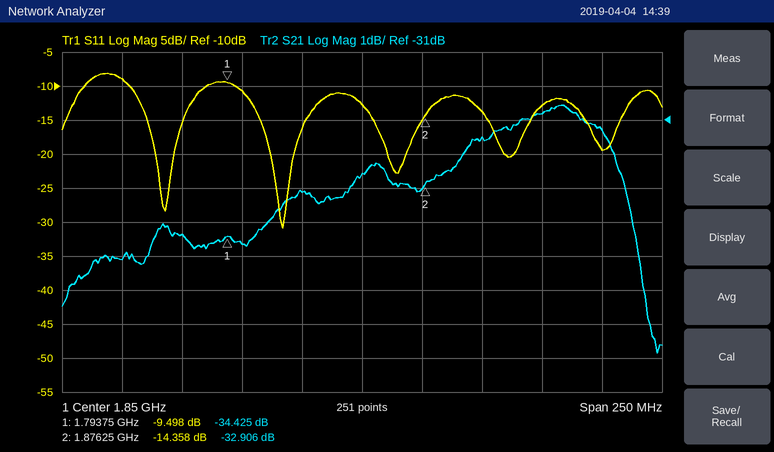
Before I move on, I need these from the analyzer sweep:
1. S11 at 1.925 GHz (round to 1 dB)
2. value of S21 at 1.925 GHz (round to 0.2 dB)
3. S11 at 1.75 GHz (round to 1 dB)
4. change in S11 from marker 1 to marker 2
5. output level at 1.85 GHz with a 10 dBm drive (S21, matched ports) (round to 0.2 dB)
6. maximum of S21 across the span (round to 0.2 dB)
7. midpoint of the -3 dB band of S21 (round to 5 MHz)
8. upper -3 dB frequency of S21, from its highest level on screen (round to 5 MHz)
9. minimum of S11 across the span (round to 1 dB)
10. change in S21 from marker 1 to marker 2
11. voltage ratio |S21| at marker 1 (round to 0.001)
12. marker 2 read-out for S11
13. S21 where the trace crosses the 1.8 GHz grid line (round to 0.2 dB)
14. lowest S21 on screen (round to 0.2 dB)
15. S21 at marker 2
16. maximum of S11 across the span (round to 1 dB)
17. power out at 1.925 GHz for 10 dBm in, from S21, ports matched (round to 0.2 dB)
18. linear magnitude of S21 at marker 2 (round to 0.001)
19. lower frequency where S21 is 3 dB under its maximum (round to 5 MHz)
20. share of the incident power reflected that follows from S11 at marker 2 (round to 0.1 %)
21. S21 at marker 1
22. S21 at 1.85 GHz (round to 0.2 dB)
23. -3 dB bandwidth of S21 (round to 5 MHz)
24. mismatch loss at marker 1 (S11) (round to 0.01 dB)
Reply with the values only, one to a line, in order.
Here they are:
-13 dB
-30.8 dB
-9 dB
-4.860 dB
-22.6 dBm
-30.6 dB
1.890 GHz
1.960 GHz
-31 dB
1.519 dB
0.019
-14.358 dB
-34.6 dB
-37.8 dB
-32.906 dB
-8 dB
-20.8 dBm
0.023
1.815 GHz
3.7 %
-34.425 dB
-32.6 dB
145 MHz
0.52 dB
